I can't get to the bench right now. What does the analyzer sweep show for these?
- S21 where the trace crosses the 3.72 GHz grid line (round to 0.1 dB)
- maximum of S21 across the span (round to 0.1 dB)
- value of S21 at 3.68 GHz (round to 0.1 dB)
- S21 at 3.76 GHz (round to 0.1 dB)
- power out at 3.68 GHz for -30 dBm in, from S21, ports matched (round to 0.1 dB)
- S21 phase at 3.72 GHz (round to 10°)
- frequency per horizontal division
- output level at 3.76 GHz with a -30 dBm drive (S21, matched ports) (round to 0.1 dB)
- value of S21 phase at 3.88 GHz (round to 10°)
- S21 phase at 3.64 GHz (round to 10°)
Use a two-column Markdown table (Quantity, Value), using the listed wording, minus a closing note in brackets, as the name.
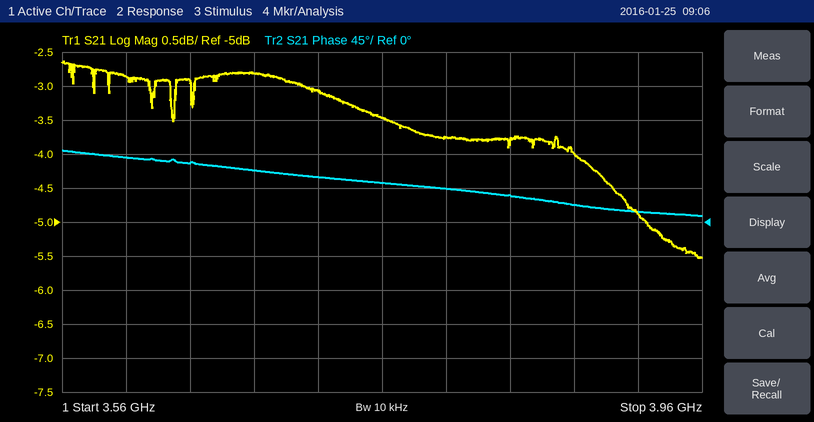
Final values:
| Quantity | Value |
|---|---|
| S21 where the trace crosses the 3.72 GHz grid line | -3.1 dB |
| maximum of S21 across the span | -2.6 dB |
| value of S21 at 3.68 GHz | -2.8 dB |
| S21 at 3.76 GHz | -3.5 dB |
| power out at 3.68 GHz for -30 dBm in, from S21, ports matched | -32.8 dBm |
| S21 phase at 3.72 GHz | 60° |
| frequency per horizontal division | 40 MHz |
| output level at 3.76 GHz with a -30 dBm drive (S21, matched ports) | -33.5 dBm |
| value of S21 phase at 3.88 GHz | 20° |
| S21 phase at 3.64 GHz | 80° |
